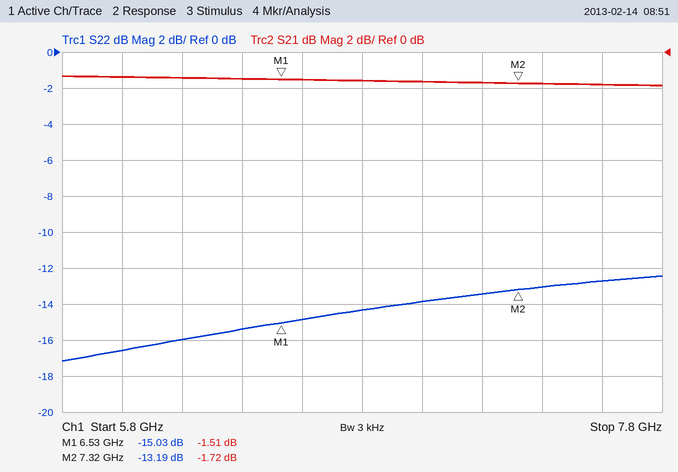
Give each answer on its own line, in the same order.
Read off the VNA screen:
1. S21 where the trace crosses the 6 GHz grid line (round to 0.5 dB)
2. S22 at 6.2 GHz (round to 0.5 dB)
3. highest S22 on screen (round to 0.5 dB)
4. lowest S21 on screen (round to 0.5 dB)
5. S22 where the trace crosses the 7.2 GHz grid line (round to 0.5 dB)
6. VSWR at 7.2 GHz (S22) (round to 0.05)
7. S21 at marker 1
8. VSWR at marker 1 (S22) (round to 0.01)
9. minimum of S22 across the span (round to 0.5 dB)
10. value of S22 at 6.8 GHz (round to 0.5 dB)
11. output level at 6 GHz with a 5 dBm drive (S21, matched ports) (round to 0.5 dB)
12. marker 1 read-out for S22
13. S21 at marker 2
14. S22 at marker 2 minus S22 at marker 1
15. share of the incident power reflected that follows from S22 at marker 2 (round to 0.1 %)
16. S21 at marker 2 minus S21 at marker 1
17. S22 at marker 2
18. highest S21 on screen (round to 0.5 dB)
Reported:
-1.5 dB
-16.0 dB
-12.5 dB
-2.0 dB
-13.5 dB
1.55
-1.51 dB
1.43
-17.0 dB
-14.5 dB
3.5 dBm
-15.03 dB
-1.72 dB
1.84 dB
4.8 %
-0.21 dB
-13.19 dB
-1.5 dB
